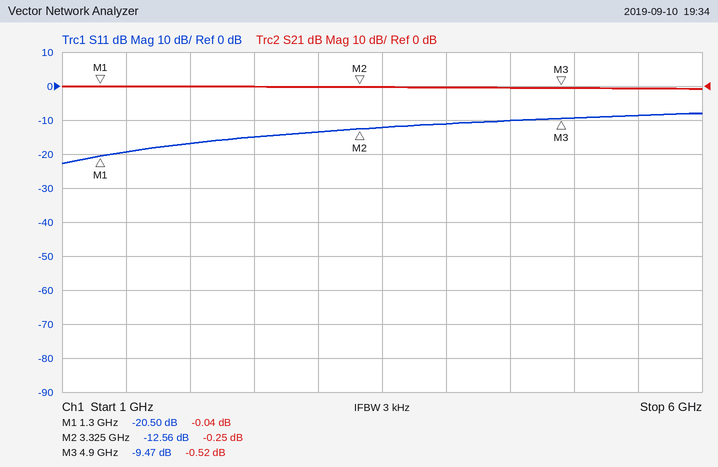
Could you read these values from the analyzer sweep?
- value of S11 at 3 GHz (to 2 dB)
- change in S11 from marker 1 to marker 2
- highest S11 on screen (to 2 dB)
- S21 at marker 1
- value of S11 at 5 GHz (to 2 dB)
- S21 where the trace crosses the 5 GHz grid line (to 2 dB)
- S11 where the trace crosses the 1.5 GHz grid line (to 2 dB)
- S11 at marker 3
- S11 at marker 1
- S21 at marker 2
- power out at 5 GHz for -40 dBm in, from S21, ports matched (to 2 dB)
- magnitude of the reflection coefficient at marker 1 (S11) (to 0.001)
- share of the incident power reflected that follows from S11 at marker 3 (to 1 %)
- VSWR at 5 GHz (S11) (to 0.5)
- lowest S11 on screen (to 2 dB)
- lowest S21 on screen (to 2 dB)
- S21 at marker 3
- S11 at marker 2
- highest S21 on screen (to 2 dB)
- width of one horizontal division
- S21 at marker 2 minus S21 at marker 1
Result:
-14 dB
7.94 dB
-8 dB
-0.04 dB
-10 dB
0 dB
-20 dB
-9.47 dB
-20.50 dB
-0.25 dB
-40 dBm
0.094
11 %
2.0
-22 dB
0 dB
-0.52 dB
-12.56 dB
0 dB
500 MHz
-0.21 dB
